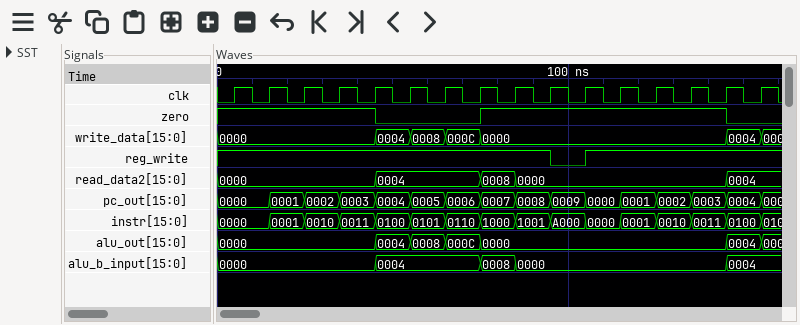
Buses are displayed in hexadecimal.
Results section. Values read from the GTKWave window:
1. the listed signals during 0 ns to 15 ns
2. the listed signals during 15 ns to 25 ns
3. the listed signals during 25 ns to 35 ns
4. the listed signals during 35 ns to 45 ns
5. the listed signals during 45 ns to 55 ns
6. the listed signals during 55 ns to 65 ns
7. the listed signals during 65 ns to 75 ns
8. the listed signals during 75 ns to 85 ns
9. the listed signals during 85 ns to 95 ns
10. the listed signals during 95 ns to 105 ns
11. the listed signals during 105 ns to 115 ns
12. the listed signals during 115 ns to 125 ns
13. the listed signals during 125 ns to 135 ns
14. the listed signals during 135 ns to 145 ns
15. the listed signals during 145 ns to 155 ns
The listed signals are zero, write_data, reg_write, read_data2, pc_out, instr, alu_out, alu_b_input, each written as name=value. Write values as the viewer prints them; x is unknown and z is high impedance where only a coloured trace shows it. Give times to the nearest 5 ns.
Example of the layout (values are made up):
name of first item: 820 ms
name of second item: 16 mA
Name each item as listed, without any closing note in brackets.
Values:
the listed signals during 0 ns to 15 ns: zero=1, write_data=0000, reg_write=1, read_data2=0000, pc_out=0000, instr=0000, alu_out=0000, alu_b_input=0000
the listed signals during 15 ns to 25 ns: zero=1, write_data=0000, reg_write=1, read_data2=0000, pc_out=0001, instr=0001, alu_out=0000, alu_b_input=0000
the listed signals during 25 ns to 35 ns: zero=1, write_data=0000, reg_write=1, read_data2=0000, pc_out=0002, instr=0010, alu_out=0000, alu_b_input=0000
the listed signals during 35 ns to 45 ns: zero=1, write_data=0000, reg_write=1, read_data2=0000, pc_out=0003, instr=0011, alu_out=0000, alu_b_input=0000
the listed signals during 45 ns to 55 ns: zero=0, write_data=0004, reg_write=1, read_data2=0004, pc_out=0004, instr=0100, alu_out=0004, alu_b_input=0004
the listed signals during 55 ns to 65 ns: zero=0, write_data=0008, reg_write=1, read_data2=0004, pc_out=0005, instr=0101, alu_out=0008, alu_b_input=0004
the listed signals during 65 ns to 75 ns: zero=0, write_data=000C, reg_write=1, read_data2=0004, pc_out=0006, instr=0110, alu_out=000C, alu_b_input=0004
the listed signals during 75 ns to 85 ns: zero=1, write_data=0000, reg_write=1, read_data2=0008, pc_out=0007, instr=1000, alu_out=0000, alu_b_input=0008
the listed signals during 85 ns to 95 ns: zero=1, write_data=0000, reg_write=1, read_data2=0000, pc_out=0008, instr=1001, alu_out=0000, alu_b_input=0000
the listed signals during 95 ns to 105 ns: zero=1, write_data=0000, reg_write=0, read_data2=0000, pc_out=0009, instr=A000, alu_out=0000, alu_b_input=0000
the listed signals during 105 ns to 115 ns: zero=1, write_data=0000, reg_write=1, read_data2=0000, pc_out=0000, instr=0000, alu_out=0000, alu_b_input=0000
the listed signals during 115 ns to 125 ns: zero=1, write_data=0000, reg_write=1, read_data2=0000, pc_out=0001, instr=0001, alu_out=0000, alu_b_input=0000
the listed signals during 125 ns to 135 ns: zero=1, write_data=0000, reg_write=1, read_data2=0000, pc_out=0002, instr=0010, alu_out=0000, alu_b_input=0000
the listed signals during 135 ns to 145 ns: zero=1, write_data=0000, reg_write=1, read_data2=0000, pc_out=0003, instr=0011, alu_out=0000, alu_b_input=0000
the listed signals during 145 ns to 155 ns: zero=0, write_data=0004, reg_write=1, read_data2=0004, pc_out=0004, instr=0100, alu_out=0004, alu_b_input=0004
